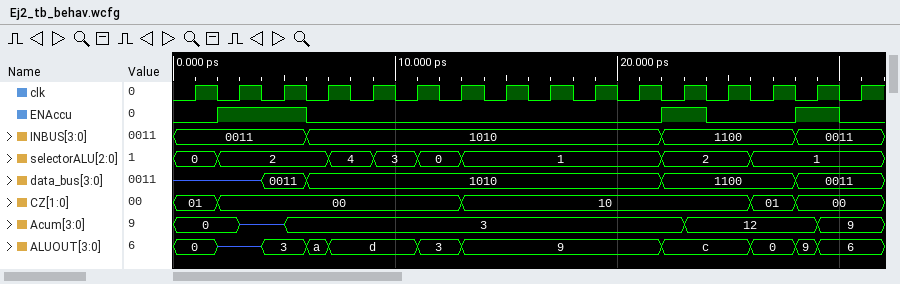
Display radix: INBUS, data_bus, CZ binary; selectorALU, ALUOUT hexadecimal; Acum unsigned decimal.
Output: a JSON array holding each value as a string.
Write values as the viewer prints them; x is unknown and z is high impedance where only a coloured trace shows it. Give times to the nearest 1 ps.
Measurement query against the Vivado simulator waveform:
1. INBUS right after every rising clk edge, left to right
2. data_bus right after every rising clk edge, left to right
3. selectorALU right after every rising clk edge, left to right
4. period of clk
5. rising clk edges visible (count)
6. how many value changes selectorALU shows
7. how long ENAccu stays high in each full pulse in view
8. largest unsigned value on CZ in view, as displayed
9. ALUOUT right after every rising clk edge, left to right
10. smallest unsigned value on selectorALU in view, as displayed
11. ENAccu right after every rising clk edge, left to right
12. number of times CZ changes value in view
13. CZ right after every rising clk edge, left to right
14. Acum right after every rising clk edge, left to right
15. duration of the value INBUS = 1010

["0011, 0011, 0011, 1010, 1010, 1010, 1010, 1010, 1010, 1010, 1010, 1100, 1100, 1100, 0011, 0011", "z, z, 0011, 1010, 1010, 1010, 1010, 1010, 1010, 1010, 1010, 1100, 1100, 1100, 0011, 0011", "0, 2, 2, 4, 3, 0, 1, 1, 1, 1, 1, 2, 2, 1, 1, 1", "2 ps", "16", "7", "4 ps, 2 ps, 2 ps", "10", "0, z, 3, d, d, 3, 9, 9, 9, 9, 9, c, c, 0, 6, 6", "0", "0 1 1 0 0 0 0 0 0 0 0 1 0 0 1 0", "4", "01, 00, 00, 00, 00, 00, 10, 10, 10, 10, 10, 10, 10, 01, 00, 00", "0, z, 3, 3, 3, 3, 3, 3, 3, 3, 3, 12, 12, 12, 9, 9", "16 ps"]
